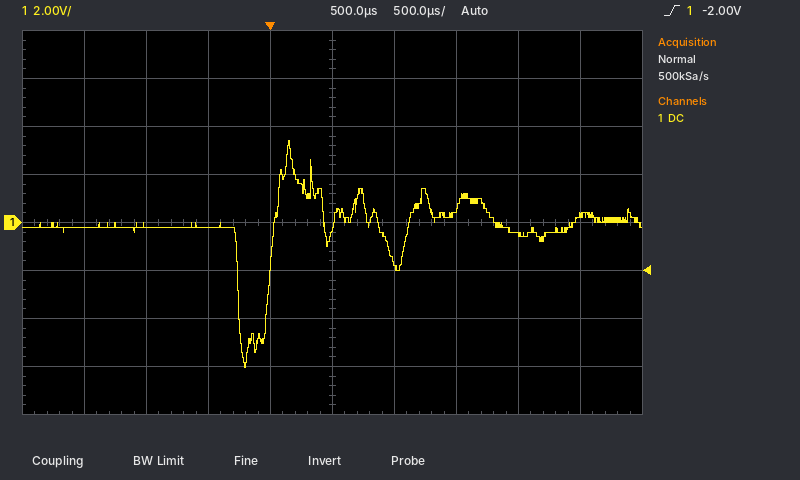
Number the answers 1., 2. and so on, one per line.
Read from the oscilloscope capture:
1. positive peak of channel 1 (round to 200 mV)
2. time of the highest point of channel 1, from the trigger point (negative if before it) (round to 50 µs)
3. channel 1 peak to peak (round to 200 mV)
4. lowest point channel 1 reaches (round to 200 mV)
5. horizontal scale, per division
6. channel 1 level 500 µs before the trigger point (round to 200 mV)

1. 3.4 V
2. +150 µs
3. 9.4 V
4. -6.0 V
5. 500 µs
6. -200 mV
